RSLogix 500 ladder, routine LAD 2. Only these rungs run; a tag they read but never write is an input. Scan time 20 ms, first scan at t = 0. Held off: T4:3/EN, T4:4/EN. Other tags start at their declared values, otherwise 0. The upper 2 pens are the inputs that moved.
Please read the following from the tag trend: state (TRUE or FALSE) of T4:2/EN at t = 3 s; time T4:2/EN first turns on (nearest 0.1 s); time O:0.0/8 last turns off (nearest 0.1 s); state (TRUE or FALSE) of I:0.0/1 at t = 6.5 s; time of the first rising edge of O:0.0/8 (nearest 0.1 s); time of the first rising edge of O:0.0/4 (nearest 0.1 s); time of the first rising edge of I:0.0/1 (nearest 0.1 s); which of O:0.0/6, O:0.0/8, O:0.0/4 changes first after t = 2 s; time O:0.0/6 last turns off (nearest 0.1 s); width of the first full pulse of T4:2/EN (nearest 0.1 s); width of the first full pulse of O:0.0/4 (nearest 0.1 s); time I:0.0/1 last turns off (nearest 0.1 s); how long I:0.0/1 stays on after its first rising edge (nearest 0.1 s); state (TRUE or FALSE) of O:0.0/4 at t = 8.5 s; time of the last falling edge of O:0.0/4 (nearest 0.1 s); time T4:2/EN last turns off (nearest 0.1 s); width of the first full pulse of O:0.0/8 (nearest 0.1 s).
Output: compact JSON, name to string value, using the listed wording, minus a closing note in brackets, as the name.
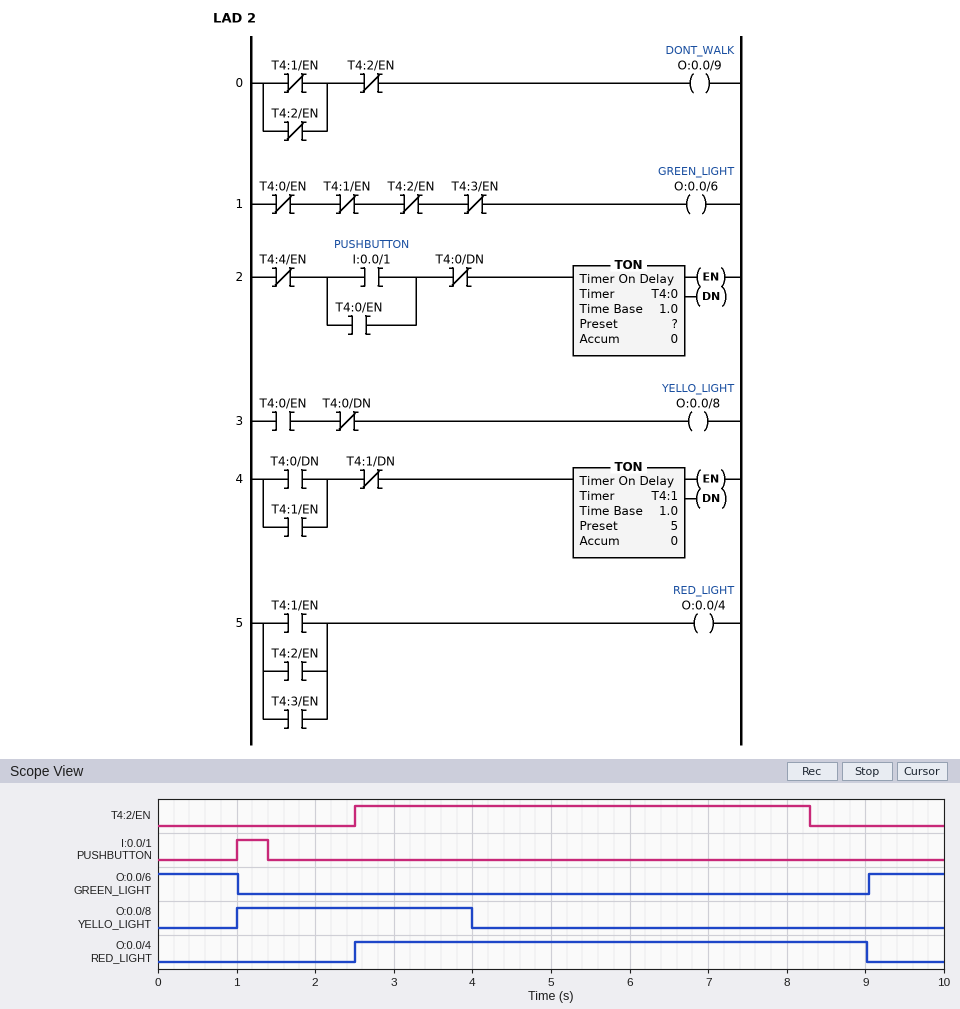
{"state (TRUE or FALSE) of T4:2/EN at t = 3 s": "TRUE", "time T4:2/EN first turns on": "2.5 s", "time O:0.0/8 last turns off": "4.0 s", "state (TRUE or FALSE) of I:0.0/1 at t = 6.5 s": "FALSE", "time of the first rising edge of O:0.0/8": "1.0 s", "time of the first rising edge of O:0.0/4": "2.5 s", "time of the first rising edge of I:0.0/1": "1.0 s", "which of O:0.0/6, O:0.0/8, O:0.0/4 changes first after t = 2 s": "O:0.0/4", "time O:0.0/6 last turns off": "1.0 s", "width of the first full pulse of T4:2/EN": "5.8 s", "width of the first full pulse of O:0.0/4": "6.5 s", "time I:0.0/1 last turns off": "1.4 s", "how long I:0.0/1 stays on after its first rising edge": "0.4 s", "state (TRUE or FALSE) of O:0.0/4 at t = 8.5 s": "TRUE", "time of the last falling edge of O:0.0/4": "9.0 s", "time T4:2/EN last turns off": "8.3 s", "width of the first full pulse of O:0.0/8": "3.0 s"}
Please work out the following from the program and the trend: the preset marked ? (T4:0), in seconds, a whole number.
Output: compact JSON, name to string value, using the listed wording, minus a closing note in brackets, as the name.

{"the preset marked ? (T4:0), in seconds, a whole number": "3 s"}
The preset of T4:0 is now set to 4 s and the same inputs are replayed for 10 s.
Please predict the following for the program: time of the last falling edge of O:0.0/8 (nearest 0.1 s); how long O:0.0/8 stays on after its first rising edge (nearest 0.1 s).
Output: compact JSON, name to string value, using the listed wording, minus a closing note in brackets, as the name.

{"time of the last falling edge of O:0.0/8": "5.0 s", "how long O:0.0/8 stays on after its first rising edge": "4.0 s"}
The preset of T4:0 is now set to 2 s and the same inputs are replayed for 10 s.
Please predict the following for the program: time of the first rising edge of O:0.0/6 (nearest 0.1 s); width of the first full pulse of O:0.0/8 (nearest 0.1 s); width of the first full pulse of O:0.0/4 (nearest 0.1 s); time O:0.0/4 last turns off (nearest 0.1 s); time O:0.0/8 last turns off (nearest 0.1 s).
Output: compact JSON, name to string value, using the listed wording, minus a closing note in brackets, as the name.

{"time of the first rising edge of O:0.0/6": "8.3 s", "width of the first full pulse of O:0.0/8": "2.0 s", "width of the first full pulse of O:0.0/4": "5.8 s", "time O:0.0/4 last turns off": "8.3 s", "time O:0.0/8 last turns off": "3.0 s"}
